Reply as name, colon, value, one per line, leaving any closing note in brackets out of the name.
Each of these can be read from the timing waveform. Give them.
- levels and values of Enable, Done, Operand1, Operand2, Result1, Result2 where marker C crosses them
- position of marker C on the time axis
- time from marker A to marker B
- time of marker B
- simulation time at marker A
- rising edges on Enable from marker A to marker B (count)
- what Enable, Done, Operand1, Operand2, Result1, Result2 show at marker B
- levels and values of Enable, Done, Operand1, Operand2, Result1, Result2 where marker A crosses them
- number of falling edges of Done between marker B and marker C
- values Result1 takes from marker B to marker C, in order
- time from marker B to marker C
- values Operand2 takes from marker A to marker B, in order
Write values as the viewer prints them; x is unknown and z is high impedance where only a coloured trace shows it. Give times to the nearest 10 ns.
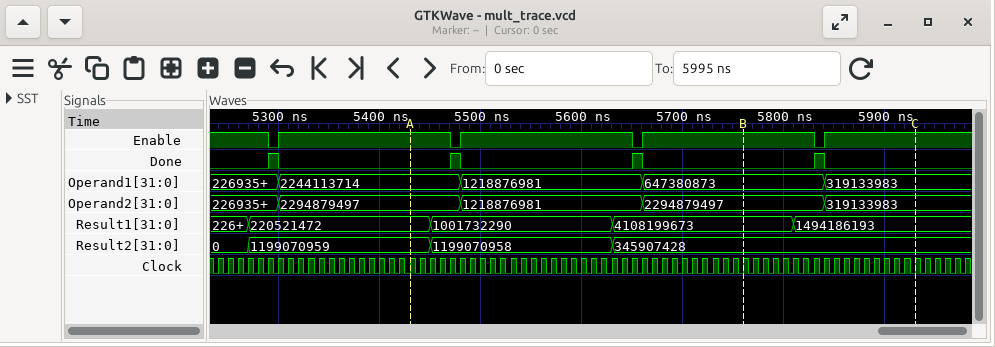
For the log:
levels and values of Enable, Done, Operand1, Operand2, Result1, Result2 where marker C crosses them: Enable=1, Done=0, Operand1=319133983, Operand2=319133983, Result1=1494186193, Result2=345907428
position of marker C on the time axis: 5930 ns
time from marker A to marker B: 330 ns
time of marker B: 5760 ns
simulation time at marker A: 5430 ns
rising edges on Enable from marker A to marker B: 2
what Enable, Done, Operand1, Operand2, Result1, Result2 show at marker B: Enable=1, Done=0, Operand1=647380873, Operand2=2294879497, Result1=4108199673, Result2=345907428
levels and values of Enable, Done, Operand1, Operand2, Result1, Result2 where marker A crosses them: Enable=1, Done=0, Operand1=2244113714, Operand2=2294879497, Result1=220521472, Result2=1199070959
number of falling edges of Done between marker B and marker C: 1
values Result1 takes from marker B to marker C, in order: 4108199673, 1494186193
time from marker B to marker C: 170 ns
values Operand2 takes from marker A to marker B, in order: 2294879497, 1218876981, 2294879497
